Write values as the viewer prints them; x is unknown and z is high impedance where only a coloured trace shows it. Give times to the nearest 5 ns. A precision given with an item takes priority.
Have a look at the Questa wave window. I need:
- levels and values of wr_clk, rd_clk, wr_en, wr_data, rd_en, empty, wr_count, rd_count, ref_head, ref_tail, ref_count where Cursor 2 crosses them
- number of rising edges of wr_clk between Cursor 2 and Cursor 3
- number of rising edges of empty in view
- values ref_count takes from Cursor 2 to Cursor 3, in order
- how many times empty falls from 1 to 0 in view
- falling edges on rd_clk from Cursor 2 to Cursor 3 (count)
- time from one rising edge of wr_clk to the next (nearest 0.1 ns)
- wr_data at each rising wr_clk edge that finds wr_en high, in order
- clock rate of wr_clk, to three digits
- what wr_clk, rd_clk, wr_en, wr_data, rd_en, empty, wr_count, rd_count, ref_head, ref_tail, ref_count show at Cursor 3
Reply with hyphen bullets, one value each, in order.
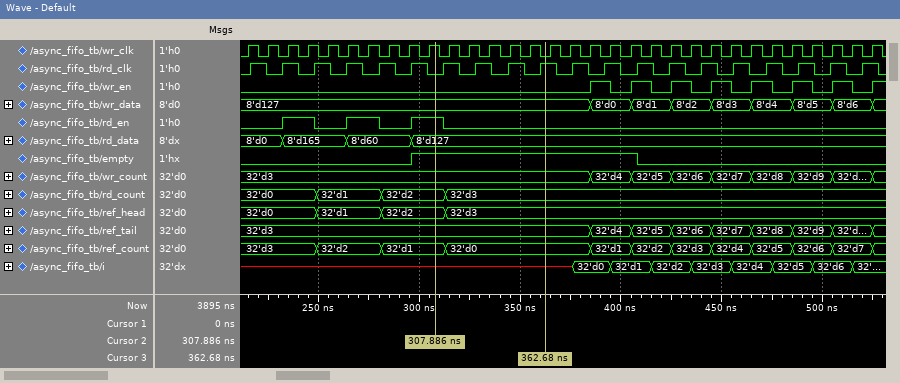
- wr_clk=1, rd_clk=0, wr_en=0, wr_data=8'd127, rd_en=1, empty=1, wr_count=32'd3, rd_count=32'd2, ref_head=32'd2, ref_tail=32'd3, ref_count=32'd1
- 5
- 1
- 32'd1, 32'd0
- 1
- 3
- 10 ns
- 8'd0, 8'd1, 8'd2, 8'd3, 8'd4, 8'd5, 8'd6
- 100 MHz
- wr_clk=0, rd_clk=1, wr_en=0, wr_data=8'd127, rd_en=0, empty=1, wr_count=32'd3, rd_count=32'd3, ref_head=32'd3, ref_tail=32'd3, ref_count=32'd0
